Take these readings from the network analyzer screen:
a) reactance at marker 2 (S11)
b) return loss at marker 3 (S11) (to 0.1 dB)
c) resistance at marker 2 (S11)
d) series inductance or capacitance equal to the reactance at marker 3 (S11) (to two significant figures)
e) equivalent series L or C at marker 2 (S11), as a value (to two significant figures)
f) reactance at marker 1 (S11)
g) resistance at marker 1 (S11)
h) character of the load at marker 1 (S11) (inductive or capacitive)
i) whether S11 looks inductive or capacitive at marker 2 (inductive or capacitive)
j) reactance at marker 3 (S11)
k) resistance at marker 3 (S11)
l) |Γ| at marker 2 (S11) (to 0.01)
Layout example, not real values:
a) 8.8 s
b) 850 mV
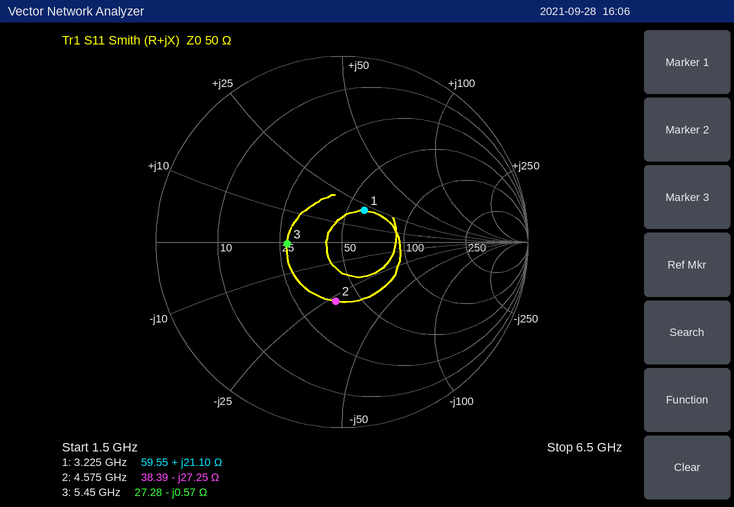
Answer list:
a) -27.25 Ω
b) 10.6 dB
c) 38.39 Ω
d) 51 pF
e) 1.3 pF
f) +21.10 Ω
g) 59.55 Ω
h) inductive
i) capacitive
j) -0.57 Ω
k) 27.28 Ω
l) 0.32
